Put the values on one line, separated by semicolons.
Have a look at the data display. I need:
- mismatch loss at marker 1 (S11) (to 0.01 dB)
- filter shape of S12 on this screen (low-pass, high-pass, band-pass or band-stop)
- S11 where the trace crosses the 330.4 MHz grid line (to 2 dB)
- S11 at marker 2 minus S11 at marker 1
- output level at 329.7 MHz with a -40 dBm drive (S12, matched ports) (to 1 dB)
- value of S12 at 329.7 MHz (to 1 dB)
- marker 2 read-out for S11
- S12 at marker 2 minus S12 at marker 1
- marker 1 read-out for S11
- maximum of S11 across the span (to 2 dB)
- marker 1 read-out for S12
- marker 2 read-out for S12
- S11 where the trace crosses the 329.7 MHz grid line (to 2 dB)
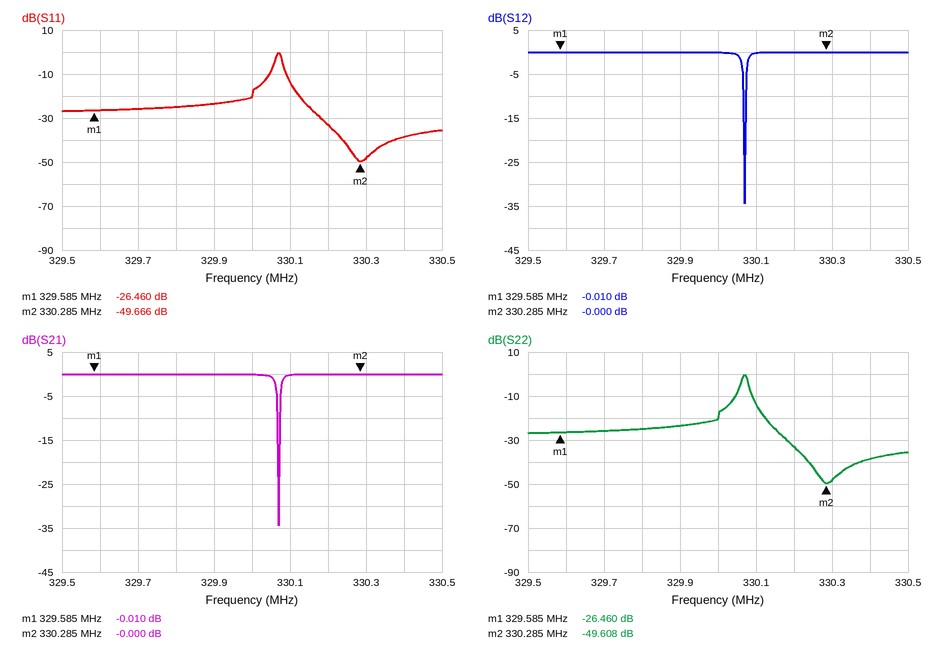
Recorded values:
0.01 dB; band-stop; -38 dB; -23.206 dB; -40 dBm; 0 dB; -49.666 dB; 0.010 dB; -26.460 dB; 0 dB; -0.010 dB; -0.000 dB; -26 dB
